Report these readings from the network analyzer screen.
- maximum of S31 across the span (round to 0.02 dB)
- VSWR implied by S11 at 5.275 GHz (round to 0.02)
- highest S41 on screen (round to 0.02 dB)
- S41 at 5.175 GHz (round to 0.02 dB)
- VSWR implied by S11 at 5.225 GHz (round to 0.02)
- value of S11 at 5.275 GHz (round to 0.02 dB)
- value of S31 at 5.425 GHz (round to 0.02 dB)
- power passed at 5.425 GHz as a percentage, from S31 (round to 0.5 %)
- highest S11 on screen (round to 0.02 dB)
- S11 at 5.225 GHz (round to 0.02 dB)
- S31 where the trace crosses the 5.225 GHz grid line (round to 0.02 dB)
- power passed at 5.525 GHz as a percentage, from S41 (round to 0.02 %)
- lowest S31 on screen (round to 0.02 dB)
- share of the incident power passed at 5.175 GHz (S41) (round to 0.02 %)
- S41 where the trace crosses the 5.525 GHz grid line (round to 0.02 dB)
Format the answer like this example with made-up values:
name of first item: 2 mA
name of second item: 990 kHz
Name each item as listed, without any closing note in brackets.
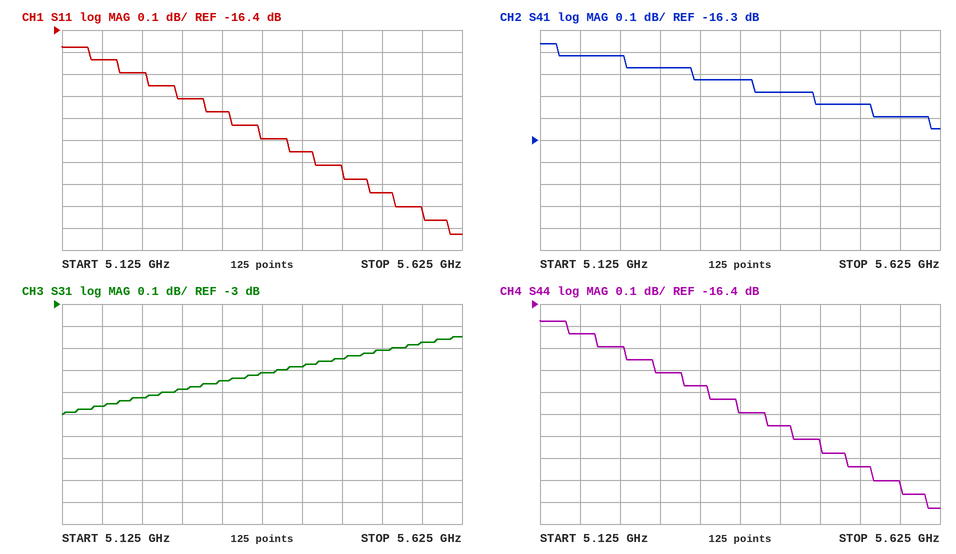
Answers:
maximum of S31 across the span: -3.14 dB
VSWR implied by S11 at 5.275 GHz: 1.34
highest S41 on screen: -15.86 dB
S41 at 5.175 GHz: -15.92 dB
VSWR implied by S11 at 5.225 GHz: 1.34
value of S11 at 5.275 GHz: -16.72 dB
value of S31 at 5.425 GHz: -3.28 dB
power passed at 5.425 GHz as a percentage, from S31: 47.0 %
highest S11 on screen: -16.48 dB
S11 at 5.225 GHz: -16.60 dB
S31 where the trace crosses the 5.225 GHz grid line: -3.42 dB
power passed at 5.525 GHz as a percentage, from S41: 2.44 %
lowest S31 on screen: -3.50 dB
share of the incident power passed at 5.175 GHz (S41): 2.56 %
S41 where the trace crosses the 5.525 GHz grid line: -16.14 dB
